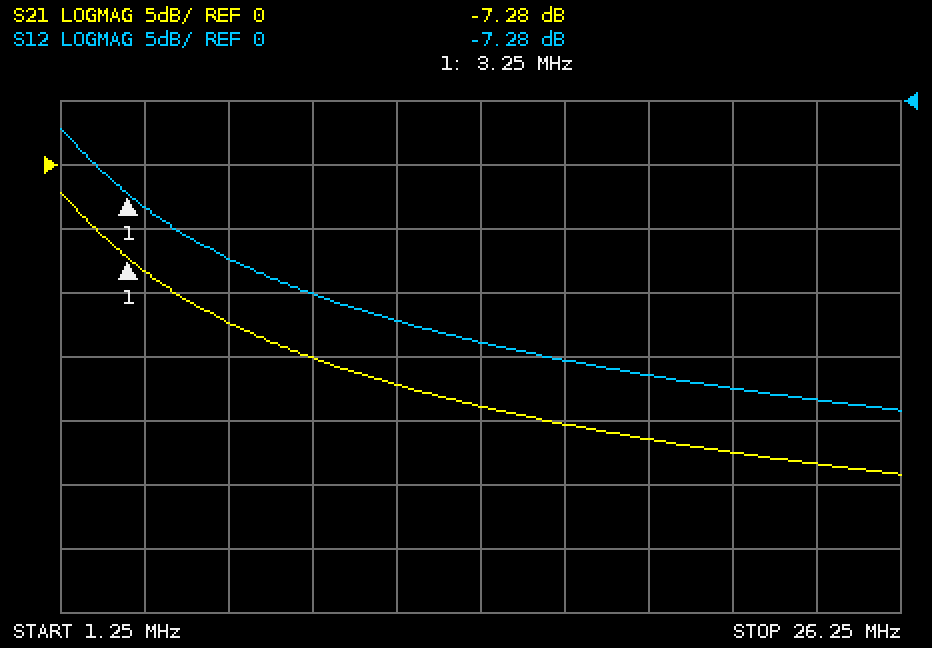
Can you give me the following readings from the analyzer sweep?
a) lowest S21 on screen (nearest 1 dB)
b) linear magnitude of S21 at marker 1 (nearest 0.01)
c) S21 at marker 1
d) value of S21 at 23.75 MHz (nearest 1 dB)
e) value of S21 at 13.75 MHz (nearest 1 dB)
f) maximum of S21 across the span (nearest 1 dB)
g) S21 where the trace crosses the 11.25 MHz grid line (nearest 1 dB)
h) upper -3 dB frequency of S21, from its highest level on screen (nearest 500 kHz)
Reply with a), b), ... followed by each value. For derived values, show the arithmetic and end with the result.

a) -24 dB
b) 10^(-7.28/20) ≈ 0.43
c) -7.28 dB
d) -23 dB
e) -19 dB
f) -2 dB
g) -17 dB
h) 2.5 MHz
